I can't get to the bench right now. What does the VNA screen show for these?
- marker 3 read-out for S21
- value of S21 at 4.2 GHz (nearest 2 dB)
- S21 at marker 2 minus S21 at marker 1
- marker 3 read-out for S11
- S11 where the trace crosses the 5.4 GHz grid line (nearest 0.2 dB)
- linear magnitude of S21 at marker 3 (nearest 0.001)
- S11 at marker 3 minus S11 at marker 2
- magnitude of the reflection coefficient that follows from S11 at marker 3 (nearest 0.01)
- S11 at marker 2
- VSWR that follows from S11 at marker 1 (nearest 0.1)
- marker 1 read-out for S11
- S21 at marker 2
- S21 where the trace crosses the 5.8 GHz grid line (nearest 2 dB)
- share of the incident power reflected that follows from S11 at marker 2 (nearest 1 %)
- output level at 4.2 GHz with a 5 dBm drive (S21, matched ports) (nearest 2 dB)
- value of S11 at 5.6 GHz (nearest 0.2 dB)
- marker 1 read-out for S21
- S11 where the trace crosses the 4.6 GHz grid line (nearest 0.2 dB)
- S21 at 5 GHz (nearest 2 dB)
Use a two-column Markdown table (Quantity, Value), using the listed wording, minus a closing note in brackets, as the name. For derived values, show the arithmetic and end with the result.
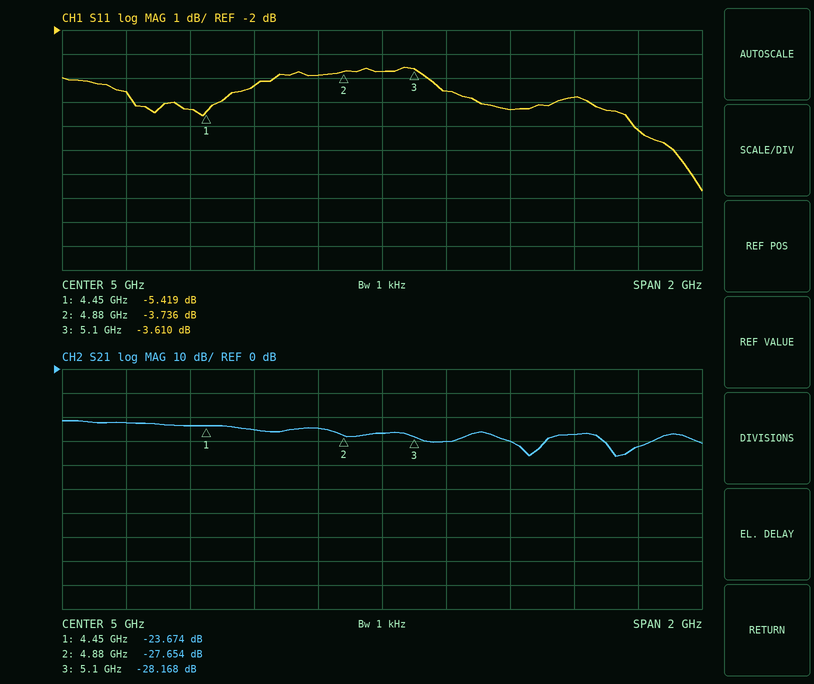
| Quantity | Value |
|---|---|
| marker 3 read-out for S21 | -28.168 dB |
| value of S21 at 4.2 GHz | -22 dB |
| S21 at marker 2 minus S21 at marker 1 | -27.654 − (-23.674) = -3.980 dB |
| marker 3 read-out for S11 | -3.610 dB |
| S11 where the trace crosses the 5.4 GHz grid line | -5.4 dB |
| linear magnitude of S21 at marker 3 | 10^(-28.168/20) ≈ 0.039 |
| S11 at marker 3 minus S11 at marker 2 | -3.61 − (-3.736) = 0.126 dB |
| magnitude of the reflection coefficient that follows from S11 at marker 3 | 10^(-3.61/20) ≈ 0.66 |
| S11 at marker 2 | -3.736 dB |
| VSWR that follows from S11 at marker 1 | (1 + 0.5359)/(1 − 0.5359) ≈ 3.3 |
| marker 1 read-out for S11 | -5.419 dB |
| S21 at marker 2 | -27.654 dB |
| S21 where the trace crosses the 5.8 GHz grid line | -32 dB |
| share of the incident power reflected that follows from S11 at marker 2 | 10^(-3.736/10) ≈ 42 % |
| output level at 4.2 GHz with a 5 dBm drive (S21, matched ports) | 5 dBm + (-22 dB) = -18 dBm |
| value of S11 at 5.6 GHz | -4.8 dB |
| marker 1 read-out for S21 | -23.674 dB |
| S11 where the trace crosses the 4.6 GHz grid line | -4.4 dB |
| S21 at 5 GHz | -26 dB |
